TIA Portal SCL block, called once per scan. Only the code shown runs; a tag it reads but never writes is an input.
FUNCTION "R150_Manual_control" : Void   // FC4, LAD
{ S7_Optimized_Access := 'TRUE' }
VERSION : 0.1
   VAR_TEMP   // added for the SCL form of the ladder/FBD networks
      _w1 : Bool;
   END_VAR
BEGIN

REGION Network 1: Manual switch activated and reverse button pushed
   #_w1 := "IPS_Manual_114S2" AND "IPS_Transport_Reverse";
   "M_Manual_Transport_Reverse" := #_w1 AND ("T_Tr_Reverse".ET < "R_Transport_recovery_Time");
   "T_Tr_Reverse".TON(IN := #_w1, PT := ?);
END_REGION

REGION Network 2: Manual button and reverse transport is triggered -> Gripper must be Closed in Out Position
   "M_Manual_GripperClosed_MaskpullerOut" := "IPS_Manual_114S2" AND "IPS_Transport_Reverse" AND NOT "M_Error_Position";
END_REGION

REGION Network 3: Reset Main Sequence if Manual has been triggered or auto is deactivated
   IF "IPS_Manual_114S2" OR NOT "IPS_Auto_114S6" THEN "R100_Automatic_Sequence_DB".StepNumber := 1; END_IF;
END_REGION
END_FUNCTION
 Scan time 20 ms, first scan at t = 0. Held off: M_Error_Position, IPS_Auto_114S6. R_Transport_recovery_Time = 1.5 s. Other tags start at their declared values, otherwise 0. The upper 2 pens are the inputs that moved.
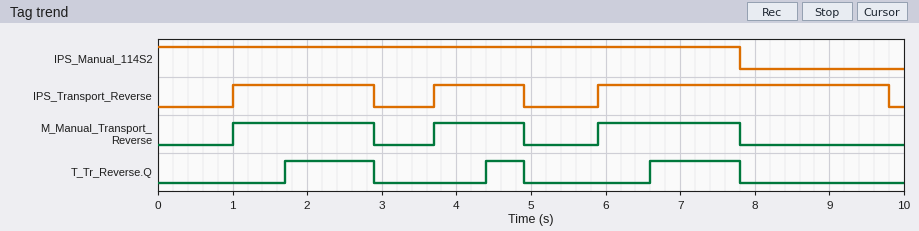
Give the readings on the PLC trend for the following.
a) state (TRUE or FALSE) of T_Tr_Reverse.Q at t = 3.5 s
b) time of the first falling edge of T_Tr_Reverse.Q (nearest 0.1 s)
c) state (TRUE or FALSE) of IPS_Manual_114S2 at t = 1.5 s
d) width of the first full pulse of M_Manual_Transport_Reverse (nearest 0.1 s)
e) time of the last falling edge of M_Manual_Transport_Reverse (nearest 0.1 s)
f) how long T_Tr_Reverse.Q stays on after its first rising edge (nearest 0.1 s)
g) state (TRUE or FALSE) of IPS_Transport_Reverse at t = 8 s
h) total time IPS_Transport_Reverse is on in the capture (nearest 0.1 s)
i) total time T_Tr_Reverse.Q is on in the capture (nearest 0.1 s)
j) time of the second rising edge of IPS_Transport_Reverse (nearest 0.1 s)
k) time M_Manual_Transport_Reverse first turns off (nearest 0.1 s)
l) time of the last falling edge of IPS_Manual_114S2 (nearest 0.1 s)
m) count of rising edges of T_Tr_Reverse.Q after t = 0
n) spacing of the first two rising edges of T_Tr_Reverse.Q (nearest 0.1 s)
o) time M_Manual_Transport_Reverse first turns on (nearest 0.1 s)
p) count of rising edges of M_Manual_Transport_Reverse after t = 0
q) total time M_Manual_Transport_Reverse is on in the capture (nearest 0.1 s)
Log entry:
FALSE
2.9 s
TRUE
1.9 s
7.8 s
1.2 s
TRUE
7.0 s
2.9 s
3.7 s
2.9 s
7.8 s
3
2.7 s
1.0 s
3
5.0 s
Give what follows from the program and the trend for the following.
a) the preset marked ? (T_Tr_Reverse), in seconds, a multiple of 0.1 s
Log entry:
0.7 s
